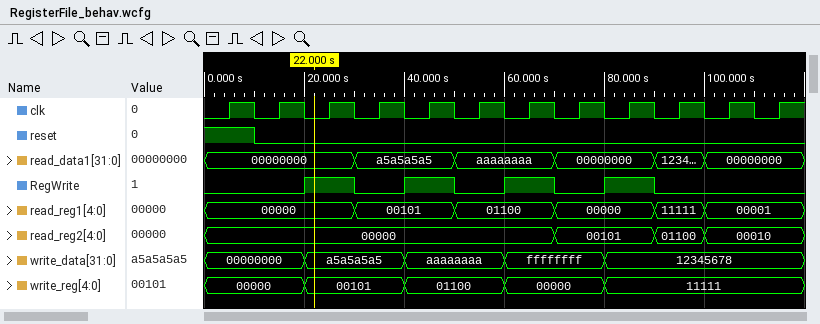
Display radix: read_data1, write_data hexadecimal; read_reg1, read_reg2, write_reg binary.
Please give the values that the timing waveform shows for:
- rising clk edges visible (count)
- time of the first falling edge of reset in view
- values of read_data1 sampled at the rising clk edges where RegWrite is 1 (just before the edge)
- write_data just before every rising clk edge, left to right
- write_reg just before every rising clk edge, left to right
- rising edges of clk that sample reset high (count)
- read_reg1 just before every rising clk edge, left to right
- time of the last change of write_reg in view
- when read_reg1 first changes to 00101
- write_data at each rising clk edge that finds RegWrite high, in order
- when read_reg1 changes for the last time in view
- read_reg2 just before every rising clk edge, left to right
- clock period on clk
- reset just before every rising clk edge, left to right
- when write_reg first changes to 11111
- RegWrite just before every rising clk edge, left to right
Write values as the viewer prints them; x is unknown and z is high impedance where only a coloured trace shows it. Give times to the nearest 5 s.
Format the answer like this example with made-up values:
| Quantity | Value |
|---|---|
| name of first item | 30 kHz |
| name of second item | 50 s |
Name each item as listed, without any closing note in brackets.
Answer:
| Quantity | Value |
|---|---|
| rising clk edges visible | 12 |
| time of the first falling edge of reset in view | 10 s |
| values of read_data1 sampled at the rising clk edges where RegWrite is 1 | 00000000, a5a5a5a5, aaaaaaaa, 00000000 |
| write_data just before every rising clk edge, left to right | 00000000, 00000000, a5a5a5a5, a5a5a5a5, aaaaaaaa, aaaaaaaa, ffffffff, ffffffff, 12345678, 12345678, 12345678, 12345678 |
| write_reg just before every rising clk edge, left to right | 00000, 00000, 00101, 00101, 01100, 01100, 00000, 00000, 11111, 11111, 11111, 11111 |
| rising edges of clk that sample reset high | 1 |
| read_reg1 just before every rising clk edge, left to right | 00000, 00000, 00000, 00101, 00101, 01100, 01100, 00000, 00000, 11111, 00001, 00001 |
| time of the last change of write_reg in view | 80 s |
| when read_reg1 first changes to 00101 | 30 s |
| write_data at each rising clk edge that finds RegWrite high, in order | a5a5a5a5, aaaaaaaa, ffffffff, 12345678 |
| when read_reg1 changes for the last time in view | 100 s |
| read_reg2 just before every rising clk edge, left to right | 00000, 00000, 00000, 00000, 00000, 00000, 00000, 00101, 00101, 01100, 00010, 00010 |
| clock period on clk | 10 s |
| reset just before every rising clk edge, left to right | 1 0 0 0 0 0 0 0 0 0 0 0 |
| when write_reg first changes to 11111 | 80 s |
| RegWrite just before every rising clk edge, left to right | 0 0 1 0 1 0 1 0 1 0 0 0 |
